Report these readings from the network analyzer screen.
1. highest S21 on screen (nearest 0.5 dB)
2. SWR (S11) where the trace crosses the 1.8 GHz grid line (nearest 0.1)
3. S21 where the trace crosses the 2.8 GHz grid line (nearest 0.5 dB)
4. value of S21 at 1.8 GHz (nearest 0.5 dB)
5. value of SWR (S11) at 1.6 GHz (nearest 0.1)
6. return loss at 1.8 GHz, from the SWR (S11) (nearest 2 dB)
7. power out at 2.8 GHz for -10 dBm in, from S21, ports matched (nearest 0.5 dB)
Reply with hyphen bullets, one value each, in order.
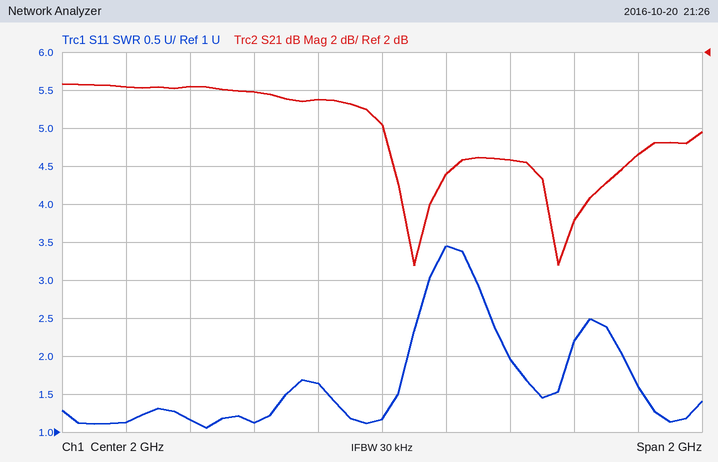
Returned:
- 0.5 dB
- 1.6
- -3.5 dB
- -0.5 dB
- 1.1
- 12 dB
- -13.5 dBm
